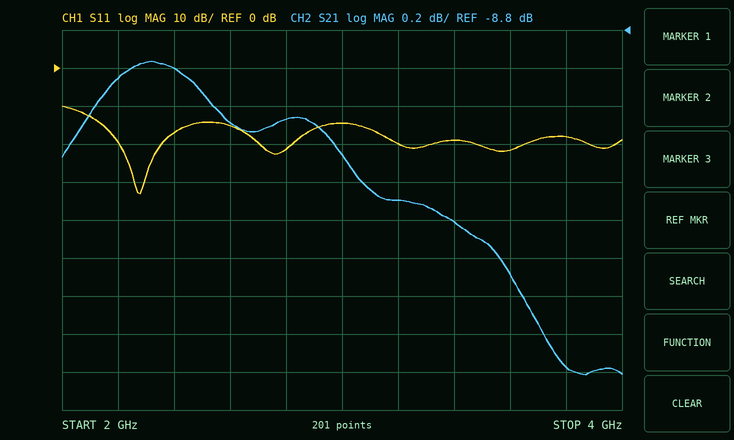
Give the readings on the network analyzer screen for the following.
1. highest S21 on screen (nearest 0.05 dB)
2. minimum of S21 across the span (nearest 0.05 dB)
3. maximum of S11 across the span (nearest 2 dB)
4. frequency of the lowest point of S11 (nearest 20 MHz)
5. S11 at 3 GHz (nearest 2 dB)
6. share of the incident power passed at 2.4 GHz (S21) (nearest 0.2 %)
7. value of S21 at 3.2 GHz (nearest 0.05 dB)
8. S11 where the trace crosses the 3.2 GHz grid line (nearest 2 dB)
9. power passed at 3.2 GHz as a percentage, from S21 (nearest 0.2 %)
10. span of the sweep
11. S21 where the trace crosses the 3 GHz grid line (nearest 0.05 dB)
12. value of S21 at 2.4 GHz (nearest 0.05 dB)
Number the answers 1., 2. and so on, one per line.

1. -8.95 dB
2. -10.60 dB
3. -10 dB
4. 2.28 GHz
5. -14 dB
6. 12.6 %
7. -9.70 dB
8. -20 dB
9. 10.8 %
10. 2 GHz
11. -9.45 dB
12. -9.00 dB
